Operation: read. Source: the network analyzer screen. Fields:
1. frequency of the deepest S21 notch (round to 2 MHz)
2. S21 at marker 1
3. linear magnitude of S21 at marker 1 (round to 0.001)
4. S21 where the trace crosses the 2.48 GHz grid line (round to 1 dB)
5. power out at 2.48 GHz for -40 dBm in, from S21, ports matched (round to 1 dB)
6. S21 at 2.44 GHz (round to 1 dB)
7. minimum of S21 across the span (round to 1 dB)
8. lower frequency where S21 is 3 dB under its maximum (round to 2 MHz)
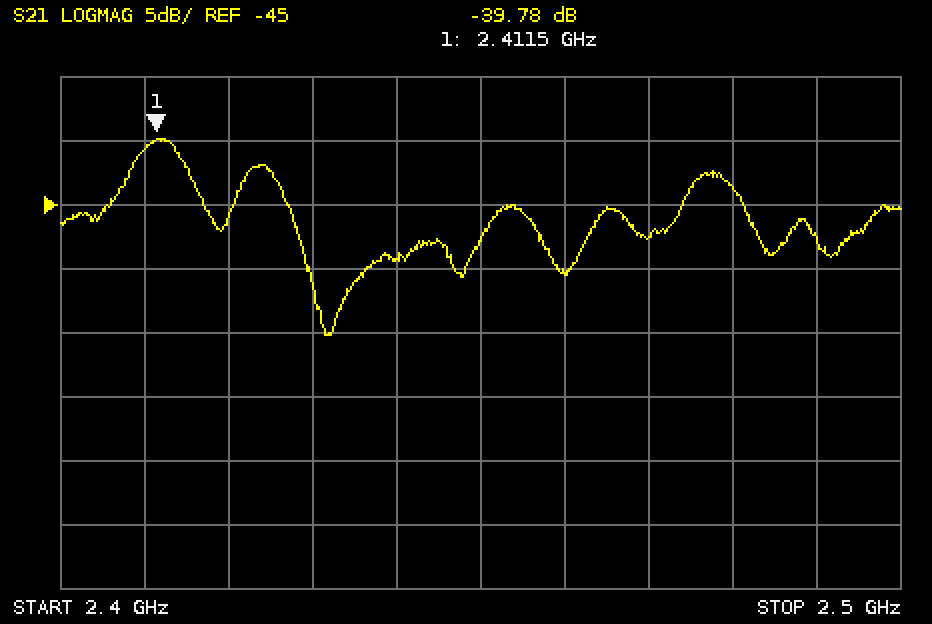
2.432 GHz
-39.78 dB
0.010
-44 dB
-84 dBm
-49 dB
-55 dB
2.408 GHz
